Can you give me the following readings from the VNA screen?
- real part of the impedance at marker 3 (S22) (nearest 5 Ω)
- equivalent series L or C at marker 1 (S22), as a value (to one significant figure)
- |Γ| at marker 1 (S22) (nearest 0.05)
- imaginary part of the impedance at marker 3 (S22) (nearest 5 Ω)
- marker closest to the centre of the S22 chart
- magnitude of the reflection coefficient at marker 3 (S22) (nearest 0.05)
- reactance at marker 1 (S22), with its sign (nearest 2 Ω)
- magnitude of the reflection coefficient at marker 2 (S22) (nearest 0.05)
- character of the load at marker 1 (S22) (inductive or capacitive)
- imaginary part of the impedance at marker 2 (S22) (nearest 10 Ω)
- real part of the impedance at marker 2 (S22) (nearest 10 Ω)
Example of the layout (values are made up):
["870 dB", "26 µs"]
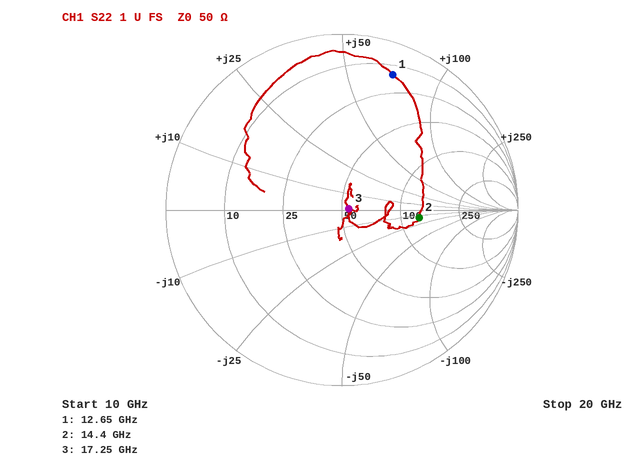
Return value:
["55 Ω", "900 pH", "0.80", "0 Ω", "marker 3", "0.05", "+70 Ω", "0.45", "inductive", "-10 Ω", "130 Ω"]
